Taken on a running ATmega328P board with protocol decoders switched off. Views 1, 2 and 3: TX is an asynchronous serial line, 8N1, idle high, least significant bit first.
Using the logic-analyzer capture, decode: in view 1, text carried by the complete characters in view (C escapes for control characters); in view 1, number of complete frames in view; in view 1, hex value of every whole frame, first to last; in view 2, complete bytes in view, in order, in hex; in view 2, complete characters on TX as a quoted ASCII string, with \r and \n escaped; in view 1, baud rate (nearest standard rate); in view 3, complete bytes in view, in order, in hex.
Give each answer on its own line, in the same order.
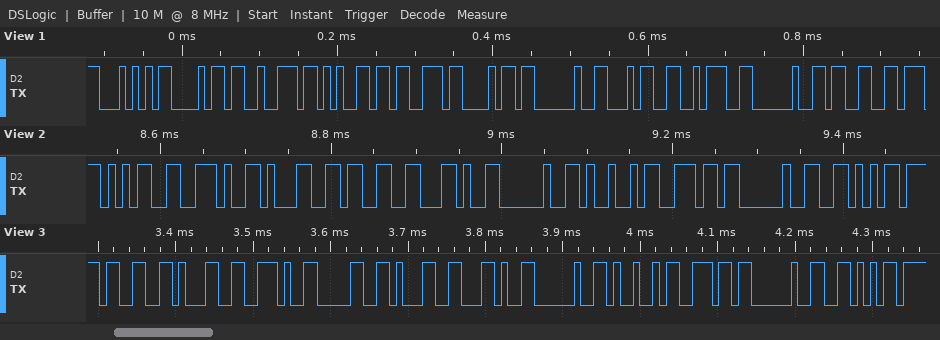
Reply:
"Thresh 4: 3"
11
0x54 0x68 0x72 0x65 0x73 0x68 0x20 0x34 0x3A 0x20 0x33
35 2E 31 33 2C 20 49 6E 20 56
"5.13, In V"
115200 baud
0x33 0x31 0x2E 0x30 0x31 0x2C 0x20 0x49 0x6E 0x20 0x56
